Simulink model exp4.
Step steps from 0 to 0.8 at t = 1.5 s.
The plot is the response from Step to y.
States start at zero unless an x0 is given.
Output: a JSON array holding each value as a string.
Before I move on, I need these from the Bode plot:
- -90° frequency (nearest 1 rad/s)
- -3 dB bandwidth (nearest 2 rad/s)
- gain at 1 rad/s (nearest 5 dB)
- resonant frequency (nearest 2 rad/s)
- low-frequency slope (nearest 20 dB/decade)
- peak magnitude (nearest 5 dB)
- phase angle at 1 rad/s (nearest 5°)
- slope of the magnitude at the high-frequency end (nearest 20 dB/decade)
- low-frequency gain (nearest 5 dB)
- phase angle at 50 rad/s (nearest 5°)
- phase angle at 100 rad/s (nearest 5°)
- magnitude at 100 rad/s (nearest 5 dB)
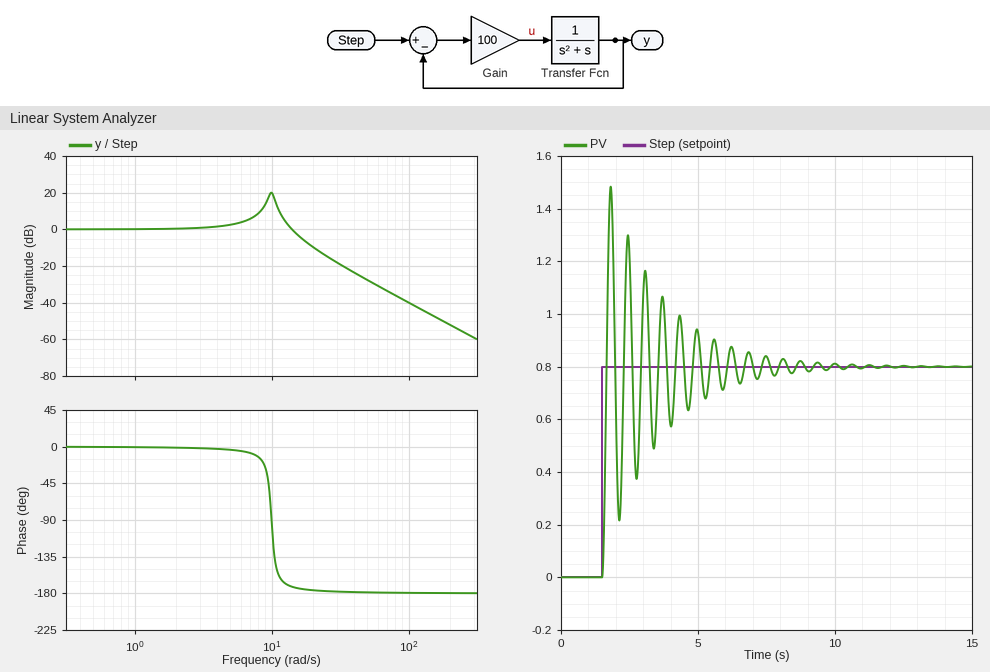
["10 rad/s", "16 rad/s", "0 dB", "10 rad/s", "0 dB/decade", "20 dB", "0°", "-40 dB/decade", "0 dB", "-180°", "-180°", "-40 dB"]
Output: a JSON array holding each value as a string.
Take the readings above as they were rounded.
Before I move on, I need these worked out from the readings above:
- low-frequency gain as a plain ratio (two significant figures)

["1.0"]
